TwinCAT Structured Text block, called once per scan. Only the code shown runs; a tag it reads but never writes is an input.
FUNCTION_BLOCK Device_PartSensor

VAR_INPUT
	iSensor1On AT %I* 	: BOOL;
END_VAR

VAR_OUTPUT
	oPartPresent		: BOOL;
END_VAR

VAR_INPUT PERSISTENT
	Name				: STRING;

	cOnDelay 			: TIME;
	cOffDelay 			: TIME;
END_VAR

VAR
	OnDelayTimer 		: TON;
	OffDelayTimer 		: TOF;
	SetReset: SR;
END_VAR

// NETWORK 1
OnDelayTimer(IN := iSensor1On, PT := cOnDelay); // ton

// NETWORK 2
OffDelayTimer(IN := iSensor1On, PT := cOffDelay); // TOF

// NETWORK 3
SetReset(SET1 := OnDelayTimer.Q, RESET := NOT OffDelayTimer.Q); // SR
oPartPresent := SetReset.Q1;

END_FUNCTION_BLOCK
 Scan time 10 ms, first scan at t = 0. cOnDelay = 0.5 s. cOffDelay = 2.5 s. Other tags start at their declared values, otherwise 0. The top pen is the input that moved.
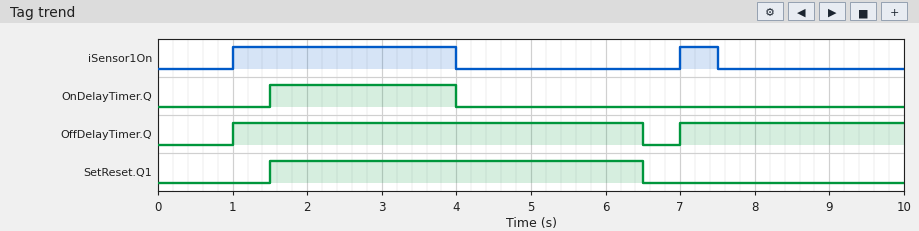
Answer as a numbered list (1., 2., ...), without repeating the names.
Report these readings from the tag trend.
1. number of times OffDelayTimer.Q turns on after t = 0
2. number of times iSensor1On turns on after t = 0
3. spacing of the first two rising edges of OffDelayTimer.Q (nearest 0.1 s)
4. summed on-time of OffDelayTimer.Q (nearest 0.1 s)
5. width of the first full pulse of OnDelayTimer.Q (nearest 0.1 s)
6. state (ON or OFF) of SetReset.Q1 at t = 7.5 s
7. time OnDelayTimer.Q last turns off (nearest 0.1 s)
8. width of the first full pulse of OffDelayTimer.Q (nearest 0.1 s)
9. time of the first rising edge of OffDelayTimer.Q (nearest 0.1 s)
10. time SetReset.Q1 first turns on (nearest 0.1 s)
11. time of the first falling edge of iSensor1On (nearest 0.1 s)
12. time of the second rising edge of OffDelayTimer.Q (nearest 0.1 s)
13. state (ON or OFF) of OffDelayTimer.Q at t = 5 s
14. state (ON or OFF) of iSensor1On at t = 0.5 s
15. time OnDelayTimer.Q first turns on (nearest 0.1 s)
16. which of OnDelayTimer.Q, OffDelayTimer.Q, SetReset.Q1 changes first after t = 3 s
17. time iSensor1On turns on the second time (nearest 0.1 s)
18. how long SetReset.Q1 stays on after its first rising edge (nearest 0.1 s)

1. 2
2. 2
3. 6.0 s
4. 8.5 s
5. 2.5 s
6. OFF
7. 4.0 s
8. 5.5 s
9. 1.0 s
10. 1.5 s
11. 4.0 s
12. 7.0 s
13. ON
14. OFF
15. 1.5 s
16. OnDelayTimer.Q
17. 7.0 s
18. 5.0 s
